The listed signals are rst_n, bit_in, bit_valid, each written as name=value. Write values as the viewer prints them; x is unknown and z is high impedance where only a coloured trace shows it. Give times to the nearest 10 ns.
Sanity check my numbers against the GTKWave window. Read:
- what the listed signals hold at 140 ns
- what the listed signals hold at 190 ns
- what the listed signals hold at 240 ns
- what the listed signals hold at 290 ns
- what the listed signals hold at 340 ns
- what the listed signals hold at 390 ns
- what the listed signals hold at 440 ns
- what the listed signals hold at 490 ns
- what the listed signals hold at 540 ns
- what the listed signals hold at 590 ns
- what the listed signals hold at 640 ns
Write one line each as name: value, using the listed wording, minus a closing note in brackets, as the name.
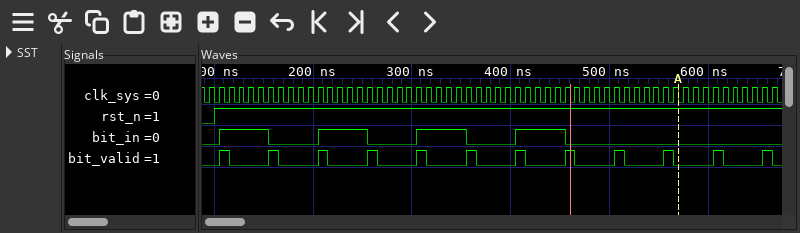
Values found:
what the listed signals hold at 140 ns: rst_n=1, bit_in=1, bit_valid=0
what the listed signals hold at 190 ns: rst_n=1, bit_in=0, bit_valid=0
what the listed signals hold at 240 ns: rst_n=1, bit_in=1, bit_valid=0
what the listed signals hold at 290 ns: rst_n=1, bit_in=0, bit_valid=0
what the listed signals hold at 340 ns: rst_n=1, bit_in=1, bit_valid=0
what the listed signals hold at 390 ns: rst_n=1, bit_in=0, bit_valid=0
what the listed signals hold at 440 ns: rst_n=1, bit_in=1, bit_valid=0
what the listed signals hold at 490 ns: rst_n=1, bit_in=0, bit_valid=0
what the listed signals hold at 540 ns: rst_n=1, bit_in=0, bit_valid=0
what the listed signals hold at 590 ns: rst_n=1, bit_in=0, bit_valid=0
what the listed signals hold at 640 ns: rst_n=1, bit_in=0, bit_valid=0
